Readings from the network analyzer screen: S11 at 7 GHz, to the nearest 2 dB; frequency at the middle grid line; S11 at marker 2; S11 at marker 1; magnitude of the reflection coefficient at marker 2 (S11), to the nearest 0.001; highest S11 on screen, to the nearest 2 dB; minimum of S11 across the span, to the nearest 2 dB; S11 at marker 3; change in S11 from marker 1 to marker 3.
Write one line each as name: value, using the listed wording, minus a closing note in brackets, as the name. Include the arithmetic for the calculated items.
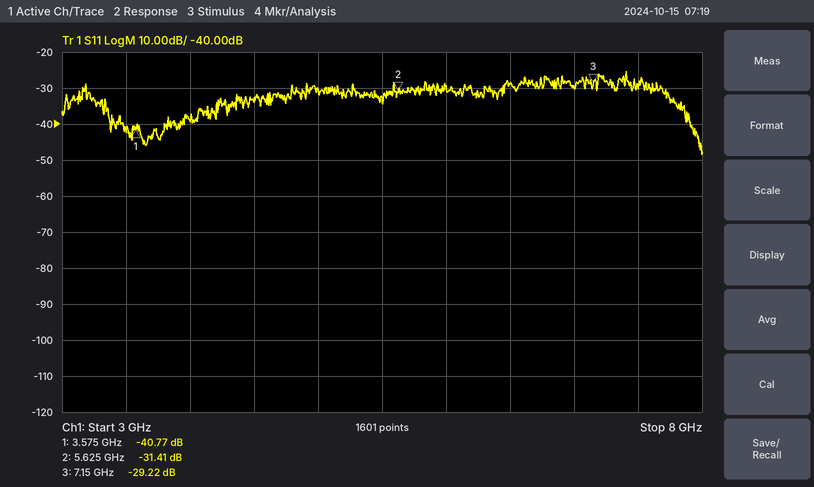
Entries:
S11 at 7 GHz, to the nearest 2 dB: -30 dB
frequency at the middle grid line: 5.5 GHz
S11 at marker 2: -31.41 dB
S11 at marker 1: -40.77 dB
magnitude of the reflection coefficient at marker 2 (S11), to the nearest 0.001: 10^(-31.41/20) ≈ 0.027
highest S11 on screen, to the nearest 2 dB: -26 dB
minimum of S11 across the span, to the nearest 2 dB: -48 dB
S11 at marker 3: -29.22 dB
change in S11 from marker 1 to marker 3: -29.22 − (-40.77) = 11.55 dB
